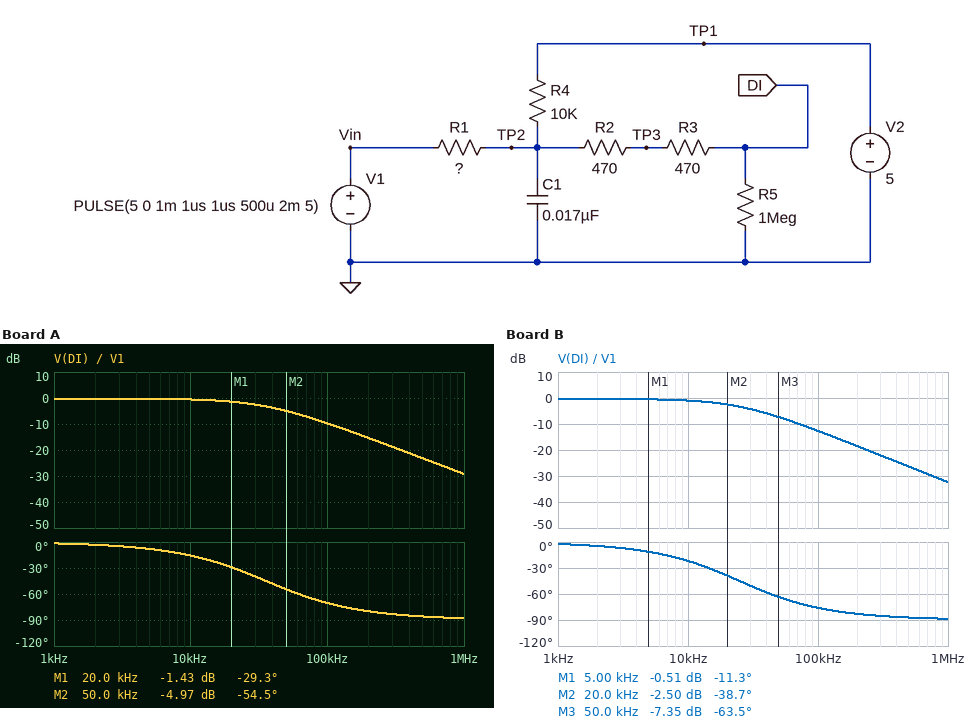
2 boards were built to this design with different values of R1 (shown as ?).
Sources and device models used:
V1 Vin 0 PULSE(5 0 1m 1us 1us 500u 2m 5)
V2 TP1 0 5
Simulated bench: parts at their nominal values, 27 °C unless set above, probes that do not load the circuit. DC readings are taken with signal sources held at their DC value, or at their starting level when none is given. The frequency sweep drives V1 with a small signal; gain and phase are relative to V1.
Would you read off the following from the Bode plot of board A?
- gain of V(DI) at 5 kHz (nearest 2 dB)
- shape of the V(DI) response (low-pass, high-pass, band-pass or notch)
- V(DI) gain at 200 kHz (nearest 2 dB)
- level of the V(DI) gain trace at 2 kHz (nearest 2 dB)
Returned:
0 dB
low-pass
-16 dB
0 dB
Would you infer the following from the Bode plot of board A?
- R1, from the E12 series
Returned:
270 Ω
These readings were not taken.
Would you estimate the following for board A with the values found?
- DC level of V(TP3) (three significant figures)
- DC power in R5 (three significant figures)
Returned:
5.00 V
24.9 µW
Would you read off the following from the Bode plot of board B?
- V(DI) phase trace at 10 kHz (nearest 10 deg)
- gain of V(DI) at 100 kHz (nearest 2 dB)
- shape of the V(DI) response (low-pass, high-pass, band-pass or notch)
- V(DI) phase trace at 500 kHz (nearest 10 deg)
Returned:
-20 deg
-12 dB
low-pass
-90 deg
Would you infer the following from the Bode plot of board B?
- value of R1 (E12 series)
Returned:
390 Ω
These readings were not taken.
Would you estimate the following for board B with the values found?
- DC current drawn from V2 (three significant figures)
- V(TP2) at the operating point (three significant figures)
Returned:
187 nA
5.00 V
